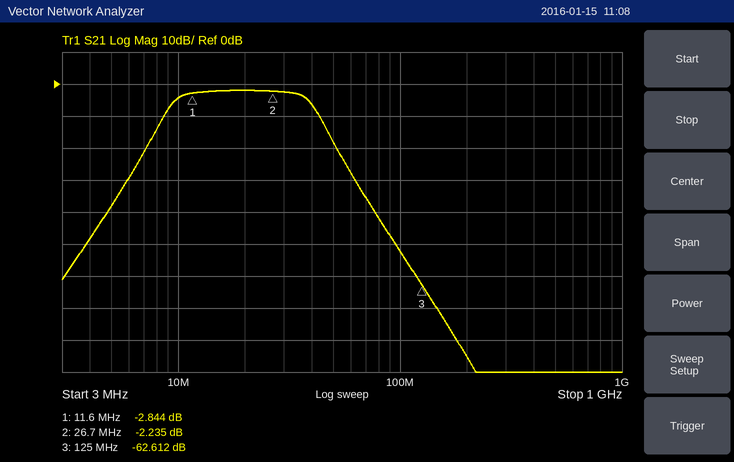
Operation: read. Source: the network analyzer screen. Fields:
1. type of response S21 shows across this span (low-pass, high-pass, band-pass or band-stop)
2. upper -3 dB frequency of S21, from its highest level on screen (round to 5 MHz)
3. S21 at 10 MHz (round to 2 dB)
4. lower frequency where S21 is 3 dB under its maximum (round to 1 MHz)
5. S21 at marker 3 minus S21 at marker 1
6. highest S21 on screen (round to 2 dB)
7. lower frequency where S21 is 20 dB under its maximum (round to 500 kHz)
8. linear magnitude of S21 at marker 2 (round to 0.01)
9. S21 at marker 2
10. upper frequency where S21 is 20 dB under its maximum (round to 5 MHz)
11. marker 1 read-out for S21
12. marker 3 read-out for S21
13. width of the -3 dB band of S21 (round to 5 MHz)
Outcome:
band-pass
40 MHz
-4 dB
10 MHz
-59.768 dB
-2 dB
7.0 MHz
0.77
-2.235 dB
55 MHz
-2.844 dB
-62.612 dB
30 MHz
